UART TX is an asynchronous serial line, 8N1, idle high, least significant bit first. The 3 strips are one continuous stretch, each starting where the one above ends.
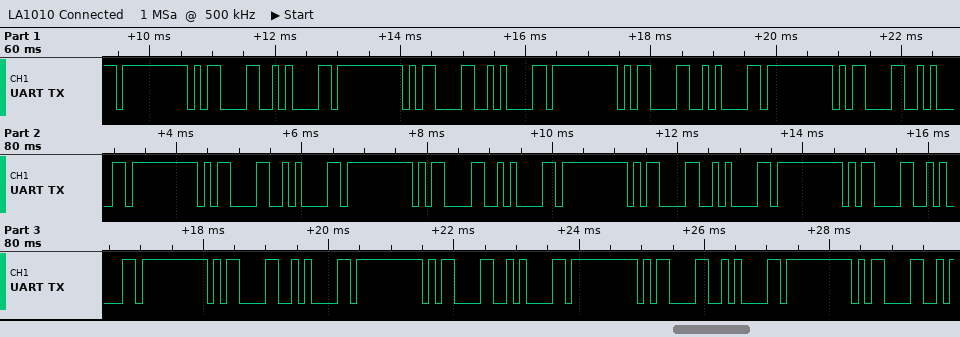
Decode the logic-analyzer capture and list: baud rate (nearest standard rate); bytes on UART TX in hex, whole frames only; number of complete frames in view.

9600 baud
FF 0D 0A FF 0D 0A FF 0D 0A FF 0D 0A FF 0D 0A FF 0D 0A FF 0D 0A FF 0D 0A FF 0D 0A FF 0D 0A FF 0D 0A FF 0D
35
